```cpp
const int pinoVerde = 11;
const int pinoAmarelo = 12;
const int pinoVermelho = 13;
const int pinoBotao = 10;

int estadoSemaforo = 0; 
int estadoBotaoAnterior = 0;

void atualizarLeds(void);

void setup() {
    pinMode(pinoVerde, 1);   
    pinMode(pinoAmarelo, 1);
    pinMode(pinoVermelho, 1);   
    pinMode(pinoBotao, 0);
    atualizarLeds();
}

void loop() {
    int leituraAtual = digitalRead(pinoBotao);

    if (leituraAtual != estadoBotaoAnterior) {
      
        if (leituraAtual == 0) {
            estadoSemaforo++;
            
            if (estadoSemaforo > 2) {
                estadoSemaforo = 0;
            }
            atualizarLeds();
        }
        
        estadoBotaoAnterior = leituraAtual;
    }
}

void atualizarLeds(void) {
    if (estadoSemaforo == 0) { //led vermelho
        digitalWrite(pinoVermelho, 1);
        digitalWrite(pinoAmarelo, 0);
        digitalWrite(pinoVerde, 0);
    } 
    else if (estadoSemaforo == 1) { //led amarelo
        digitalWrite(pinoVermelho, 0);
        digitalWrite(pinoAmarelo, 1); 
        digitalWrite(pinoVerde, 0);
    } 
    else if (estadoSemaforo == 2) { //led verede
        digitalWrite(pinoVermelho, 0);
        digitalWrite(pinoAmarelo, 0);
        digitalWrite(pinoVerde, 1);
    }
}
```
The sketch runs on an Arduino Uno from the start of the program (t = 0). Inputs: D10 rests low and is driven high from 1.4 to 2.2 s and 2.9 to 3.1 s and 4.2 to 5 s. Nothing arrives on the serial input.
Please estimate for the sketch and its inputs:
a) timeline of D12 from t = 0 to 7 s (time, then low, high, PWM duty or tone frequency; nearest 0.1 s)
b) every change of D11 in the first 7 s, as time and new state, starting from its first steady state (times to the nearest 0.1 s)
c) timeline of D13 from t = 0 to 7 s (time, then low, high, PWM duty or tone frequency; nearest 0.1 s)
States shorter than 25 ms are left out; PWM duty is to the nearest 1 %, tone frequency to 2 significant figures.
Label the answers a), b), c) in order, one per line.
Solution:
a) 0 s low; 2.2 s high; 3.1 s low
b) 0 s low; 3.1 s high; 5 s low
c) 0 s high; 2.2 s low; 5 s high
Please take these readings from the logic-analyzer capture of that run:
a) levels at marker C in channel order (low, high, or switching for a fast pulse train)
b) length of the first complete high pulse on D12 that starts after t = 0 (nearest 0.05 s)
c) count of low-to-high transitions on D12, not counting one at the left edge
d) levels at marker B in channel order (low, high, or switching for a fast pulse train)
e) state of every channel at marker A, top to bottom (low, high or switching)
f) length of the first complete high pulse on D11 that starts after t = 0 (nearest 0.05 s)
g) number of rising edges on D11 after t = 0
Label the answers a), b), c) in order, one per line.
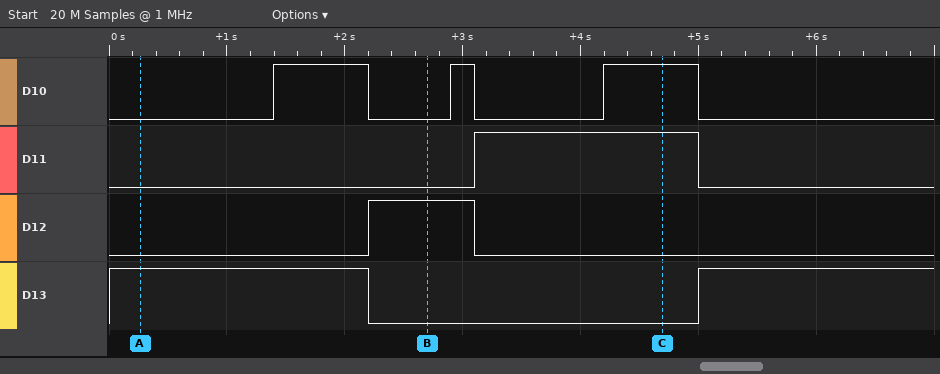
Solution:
a) D10 high, D11 high, D12 low, D13 low
b) 0.90 s
c) 1
d) D10 low, D11 low, D12 high, D13 low
e) D10 low, D11 low, D12 low, D13 high
f) 1.90 s
g) 1
